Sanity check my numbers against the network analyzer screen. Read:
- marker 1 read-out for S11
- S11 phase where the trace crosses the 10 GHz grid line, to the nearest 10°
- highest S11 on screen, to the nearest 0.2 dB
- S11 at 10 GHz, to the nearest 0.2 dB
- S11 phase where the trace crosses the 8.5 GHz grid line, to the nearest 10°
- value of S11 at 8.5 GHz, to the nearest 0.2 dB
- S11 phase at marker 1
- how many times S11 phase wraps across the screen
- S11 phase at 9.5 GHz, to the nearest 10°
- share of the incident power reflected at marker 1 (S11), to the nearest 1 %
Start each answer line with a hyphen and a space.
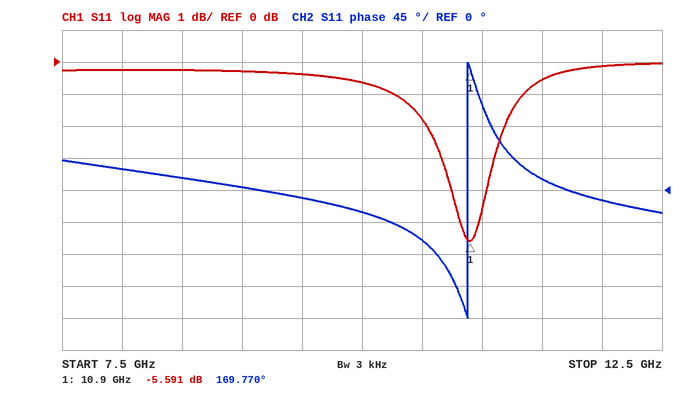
- -5.591 dB
- -30°
- 0.0 dB
- -0.6 dB
- 20°
- -0.2 dB
- 169.770°
- 1
- -10°
- 28 %
